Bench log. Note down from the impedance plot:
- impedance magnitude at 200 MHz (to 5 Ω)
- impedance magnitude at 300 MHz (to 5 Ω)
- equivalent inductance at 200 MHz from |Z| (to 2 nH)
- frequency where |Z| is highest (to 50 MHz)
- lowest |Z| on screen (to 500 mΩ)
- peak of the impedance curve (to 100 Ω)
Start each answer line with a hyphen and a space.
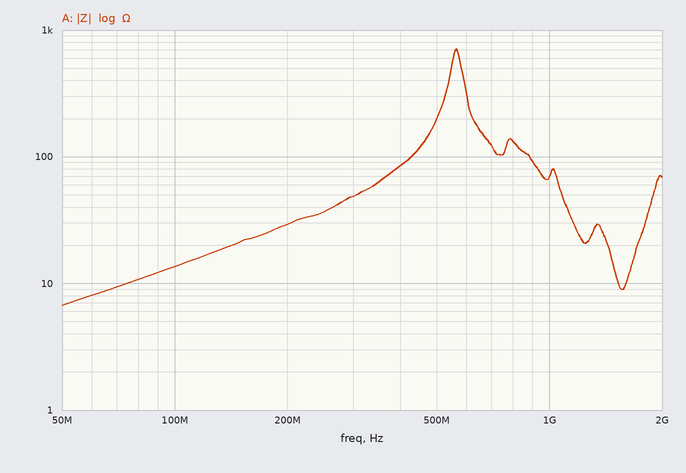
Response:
- 30 Ω
- 50 Ω
- 24 nH
- 550 MHz
- 6.5 Ω
- 700 Ω
